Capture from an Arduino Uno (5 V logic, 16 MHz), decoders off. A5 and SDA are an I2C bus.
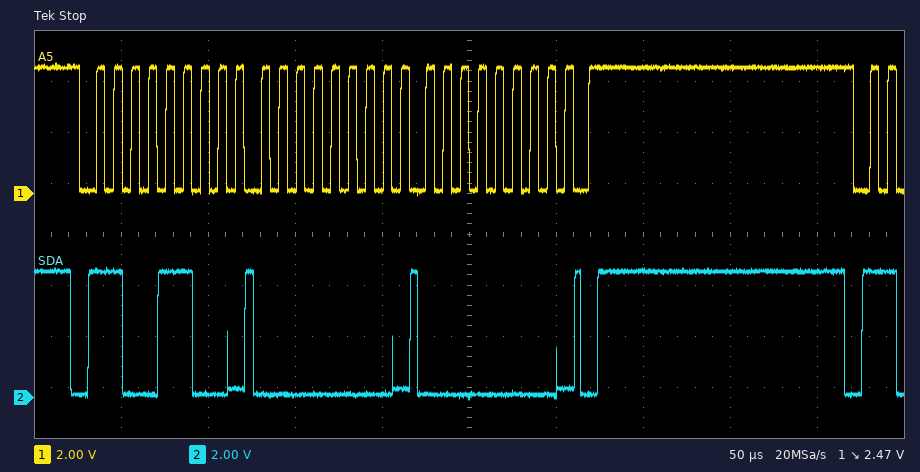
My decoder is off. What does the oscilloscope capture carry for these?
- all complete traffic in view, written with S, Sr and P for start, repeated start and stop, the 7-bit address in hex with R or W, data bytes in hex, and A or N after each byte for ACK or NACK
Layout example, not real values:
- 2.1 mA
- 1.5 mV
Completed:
- S 66W A 00 A 00 A P
